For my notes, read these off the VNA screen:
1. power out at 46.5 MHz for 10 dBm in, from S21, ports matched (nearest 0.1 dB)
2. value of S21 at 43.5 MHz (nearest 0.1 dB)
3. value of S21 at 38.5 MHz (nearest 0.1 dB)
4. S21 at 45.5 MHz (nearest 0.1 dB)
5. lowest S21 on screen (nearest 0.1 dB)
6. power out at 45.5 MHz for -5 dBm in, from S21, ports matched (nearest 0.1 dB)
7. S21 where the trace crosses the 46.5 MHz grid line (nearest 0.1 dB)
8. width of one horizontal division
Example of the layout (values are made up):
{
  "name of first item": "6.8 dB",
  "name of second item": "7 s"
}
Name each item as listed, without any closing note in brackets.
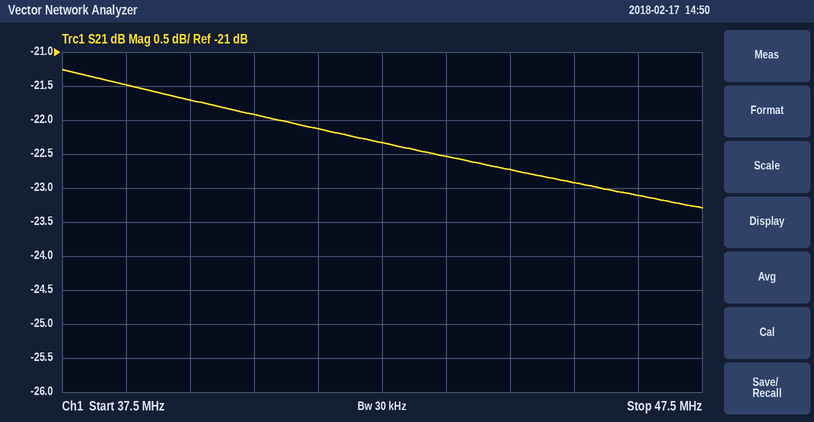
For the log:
{
  "power out at 46.5 MHz for 10 dBm in, from S21, ports matched": "-13.1 dBm",
  "value of S21 at 43.5 MHz": "-22.5 dB",
  "value of S21 at 38.5 MHz": "-21.5 dB",
  "S21 at 45.5 MHz": "-22.9 dB",
  "lowest S21 on screen": "-23.3 dB",
  "power out at 45.5 MHz for -5 dBm in, from S21, ports matched": "-27.9 dBm",
  "S21 where the trace crosses the 46.5 MHz grid line": "-23.1 dB",
  "width of one horizontal division": "1 MHz"
}
